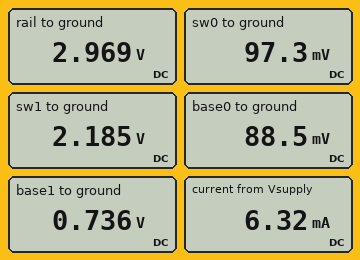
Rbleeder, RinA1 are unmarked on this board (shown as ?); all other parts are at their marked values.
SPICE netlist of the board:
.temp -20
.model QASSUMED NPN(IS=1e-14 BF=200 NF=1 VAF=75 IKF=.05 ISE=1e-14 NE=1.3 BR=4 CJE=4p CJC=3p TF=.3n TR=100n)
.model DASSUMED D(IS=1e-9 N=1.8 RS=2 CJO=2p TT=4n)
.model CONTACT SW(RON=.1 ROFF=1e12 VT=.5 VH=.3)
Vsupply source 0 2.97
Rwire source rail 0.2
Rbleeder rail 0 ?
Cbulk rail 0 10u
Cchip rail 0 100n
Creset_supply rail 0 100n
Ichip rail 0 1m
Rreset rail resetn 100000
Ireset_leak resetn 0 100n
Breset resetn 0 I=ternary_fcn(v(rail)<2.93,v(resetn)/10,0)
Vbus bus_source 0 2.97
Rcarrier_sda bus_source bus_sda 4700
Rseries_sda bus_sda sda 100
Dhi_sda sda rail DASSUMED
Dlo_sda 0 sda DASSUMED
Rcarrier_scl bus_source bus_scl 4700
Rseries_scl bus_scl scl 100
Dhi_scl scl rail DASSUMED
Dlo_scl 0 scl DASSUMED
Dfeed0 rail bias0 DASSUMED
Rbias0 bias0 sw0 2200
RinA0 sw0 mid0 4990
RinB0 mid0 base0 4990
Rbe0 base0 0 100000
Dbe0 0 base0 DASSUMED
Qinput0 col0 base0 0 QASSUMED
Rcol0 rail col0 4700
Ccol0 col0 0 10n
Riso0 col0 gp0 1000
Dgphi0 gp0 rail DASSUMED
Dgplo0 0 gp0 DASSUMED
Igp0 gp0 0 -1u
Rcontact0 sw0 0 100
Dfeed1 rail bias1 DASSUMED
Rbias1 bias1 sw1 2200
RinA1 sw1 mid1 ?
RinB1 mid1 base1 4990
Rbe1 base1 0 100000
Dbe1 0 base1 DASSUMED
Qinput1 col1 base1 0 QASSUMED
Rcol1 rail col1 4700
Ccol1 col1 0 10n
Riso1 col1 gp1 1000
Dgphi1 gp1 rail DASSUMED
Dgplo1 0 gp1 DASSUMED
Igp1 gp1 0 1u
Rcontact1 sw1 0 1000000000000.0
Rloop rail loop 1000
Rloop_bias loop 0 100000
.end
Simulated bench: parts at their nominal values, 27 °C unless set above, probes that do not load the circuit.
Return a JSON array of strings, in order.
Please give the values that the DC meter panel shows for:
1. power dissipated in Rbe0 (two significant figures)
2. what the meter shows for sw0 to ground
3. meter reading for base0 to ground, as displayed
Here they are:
["78 nW", "97.3 mV", "88.5 mV"]
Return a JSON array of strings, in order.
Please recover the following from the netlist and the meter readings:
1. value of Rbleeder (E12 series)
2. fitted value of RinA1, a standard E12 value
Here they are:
["820 Ω", "15 kΩ"]
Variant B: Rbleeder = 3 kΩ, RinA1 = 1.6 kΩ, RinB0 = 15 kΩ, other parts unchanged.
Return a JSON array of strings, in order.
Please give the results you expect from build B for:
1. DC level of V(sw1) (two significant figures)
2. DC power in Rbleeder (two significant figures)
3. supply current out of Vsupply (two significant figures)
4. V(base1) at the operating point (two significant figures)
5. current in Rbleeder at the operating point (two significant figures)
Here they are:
["1.9 V", "2.9 mW", "3.8 mA", "750 mV", "990 µA"]
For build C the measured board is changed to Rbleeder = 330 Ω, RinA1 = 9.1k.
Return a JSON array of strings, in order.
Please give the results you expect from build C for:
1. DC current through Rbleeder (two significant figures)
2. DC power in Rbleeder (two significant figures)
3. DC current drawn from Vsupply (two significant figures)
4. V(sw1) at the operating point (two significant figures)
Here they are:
["9.0 mA", "27 mW", "12 mA", "2.1 V"]
